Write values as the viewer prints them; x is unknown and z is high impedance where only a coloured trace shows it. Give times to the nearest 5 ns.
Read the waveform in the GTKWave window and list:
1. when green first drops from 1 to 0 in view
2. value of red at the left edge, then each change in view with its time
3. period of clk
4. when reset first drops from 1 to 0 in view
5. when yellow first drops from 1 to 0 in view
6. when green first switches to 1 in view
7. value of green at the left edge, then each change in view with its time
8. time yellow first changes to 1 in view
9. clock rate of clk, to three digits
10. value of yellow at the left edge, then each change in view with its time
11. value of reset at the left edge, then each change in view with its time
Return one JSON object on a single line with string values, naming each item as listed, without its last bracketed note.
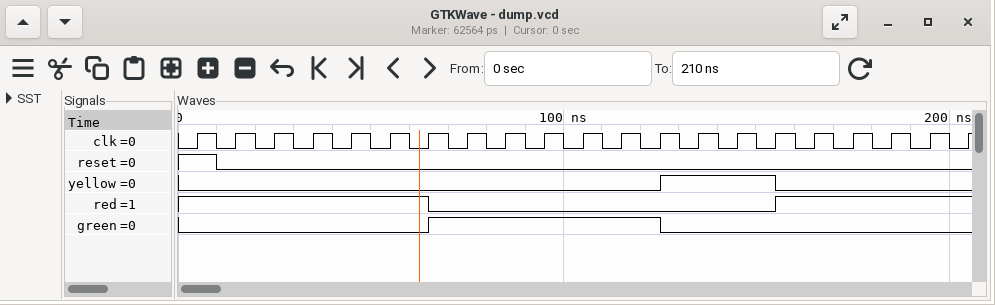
{"when green first drops from 1 to 0 in view": "125 ns", "value of red at the left edge, then each change in view with its time": "1, 0 at 65 ns, 1 at 155 ns", "period of clk": "10 ns", "when reset first drops from 1 to 0 in view": "10 ns", "when yellow first drops from 1 to 0 in view": "155 ns", "when green first switches to 1 in view": "65 ns", "value of green at the left edge, then each change in view with its time": "0, 1 at 65 ns, 0 at 125 ns", "time yellow first changes to 1 in view": "125 ns", "clock rate of clk, to three digits": "100 MHz", "value of yellow at the left edge, then each change in view with its time": "0, 1 at 125 ns, 0 at 155 ns", "value of reset at the left edge, then each change in view with its time": "1, 0 at 10 ns"}
